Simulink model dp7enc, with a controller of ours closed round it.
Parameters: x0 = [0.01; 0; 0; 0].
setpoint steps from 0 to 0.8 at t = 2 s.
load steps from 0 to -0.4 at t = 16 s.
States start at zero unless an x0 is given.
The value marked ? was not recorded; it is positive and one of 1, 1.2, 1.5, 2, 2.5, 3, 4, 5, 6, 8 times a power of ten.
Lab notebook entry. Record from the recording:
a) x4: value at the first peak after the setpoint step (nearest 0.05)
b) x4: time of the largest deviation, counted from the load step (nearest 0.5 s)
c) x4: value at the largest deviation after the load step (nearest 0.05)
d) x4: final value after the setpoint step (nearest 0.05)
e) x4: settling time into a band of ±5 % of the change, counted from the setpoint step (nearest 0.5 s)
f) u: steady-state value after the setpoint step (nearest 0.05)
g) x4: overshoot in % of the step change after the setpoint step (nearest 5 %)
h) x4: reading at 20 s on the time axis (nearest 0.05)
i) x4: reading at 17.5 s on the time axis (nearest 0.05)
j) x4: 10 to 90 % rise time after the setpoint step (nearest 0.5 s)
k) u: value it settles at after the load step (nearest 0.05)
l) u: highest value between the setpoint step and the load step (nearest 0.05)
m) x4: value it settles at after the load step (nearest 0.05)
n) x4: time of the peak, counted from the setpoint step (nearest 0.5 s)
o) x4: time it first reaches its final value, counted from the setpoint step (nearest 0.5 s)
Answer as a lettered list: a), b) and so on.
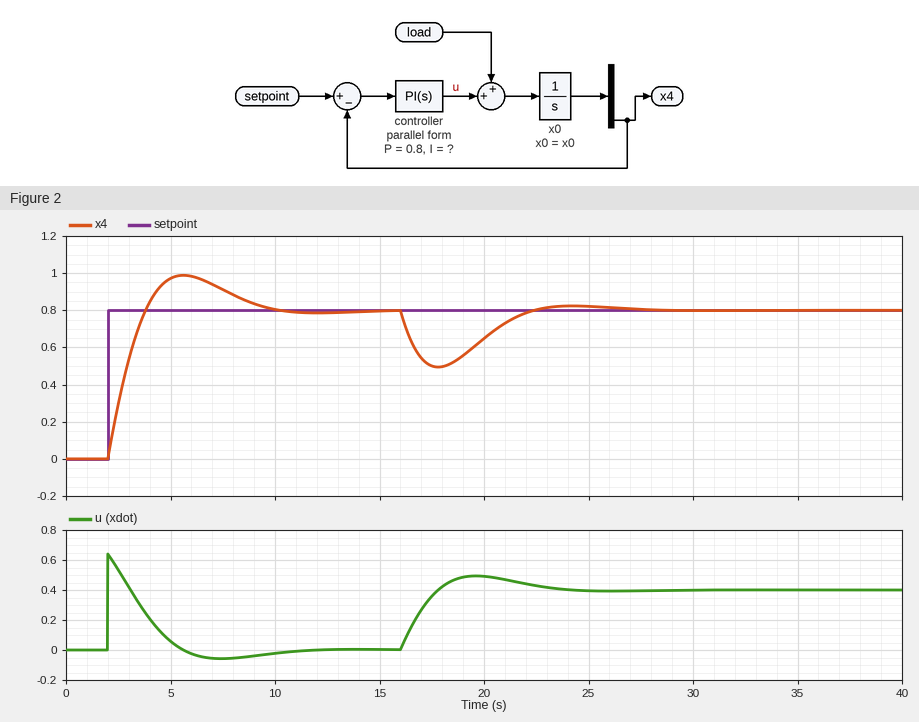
a) 1.00
b) 2.0 s
c) 0.50
d) 0.80
e) 7.0 s
f) 0.00
g) 25 %
h) 0.65
i) 0.50
j) 1.5 s
k) 0.40
l) 0.65
m) 0.80
n) 3.5 s
o) 2.0 s
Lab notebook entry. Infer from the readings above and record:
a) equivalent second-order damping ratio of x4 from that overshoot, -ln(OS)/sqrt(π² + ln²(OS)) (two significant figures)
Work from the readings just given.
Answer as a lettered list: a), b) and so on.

a) 0.40
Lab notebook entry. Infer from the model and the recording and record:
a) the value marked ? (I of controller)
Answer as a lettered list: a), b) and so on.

a) 0.4
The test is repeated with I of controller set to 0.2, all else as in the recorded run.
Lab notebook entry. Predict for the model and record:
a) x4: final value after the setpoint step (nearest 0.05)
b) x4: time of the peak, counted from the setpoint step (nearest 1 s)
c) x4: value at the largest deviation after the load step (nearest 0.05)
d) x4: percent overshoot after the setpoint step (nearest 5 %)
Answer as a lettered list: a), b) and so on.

a) 0.80
b) 5 s
c) 0.45
d) 15 %
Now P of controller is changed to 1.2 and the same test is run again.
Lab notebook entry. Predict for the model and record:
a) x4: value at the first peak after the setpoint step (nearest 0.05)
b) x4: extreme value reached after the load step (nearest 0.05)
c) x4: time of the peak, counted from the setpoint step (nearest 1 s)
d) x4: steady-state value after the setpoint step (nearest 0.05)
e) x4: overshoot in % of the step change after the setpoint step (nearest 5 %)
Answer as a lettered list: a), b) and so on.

a) 0.90
b) 0.55
c) 3 s
d) 0.80
e) 15 %
